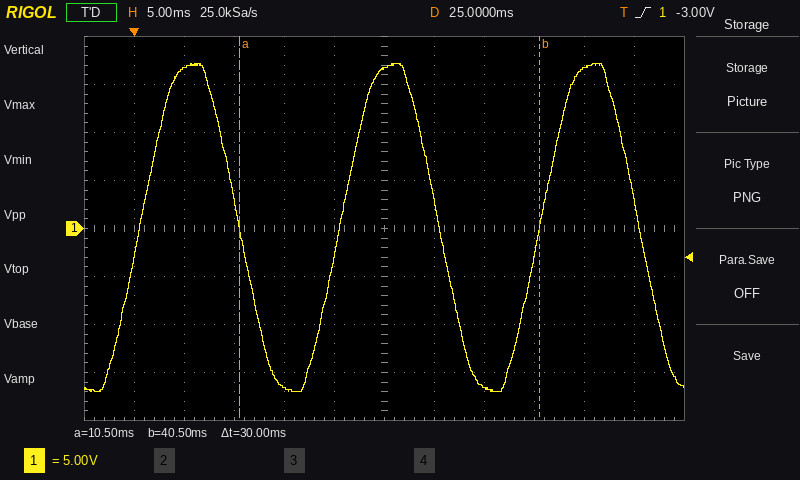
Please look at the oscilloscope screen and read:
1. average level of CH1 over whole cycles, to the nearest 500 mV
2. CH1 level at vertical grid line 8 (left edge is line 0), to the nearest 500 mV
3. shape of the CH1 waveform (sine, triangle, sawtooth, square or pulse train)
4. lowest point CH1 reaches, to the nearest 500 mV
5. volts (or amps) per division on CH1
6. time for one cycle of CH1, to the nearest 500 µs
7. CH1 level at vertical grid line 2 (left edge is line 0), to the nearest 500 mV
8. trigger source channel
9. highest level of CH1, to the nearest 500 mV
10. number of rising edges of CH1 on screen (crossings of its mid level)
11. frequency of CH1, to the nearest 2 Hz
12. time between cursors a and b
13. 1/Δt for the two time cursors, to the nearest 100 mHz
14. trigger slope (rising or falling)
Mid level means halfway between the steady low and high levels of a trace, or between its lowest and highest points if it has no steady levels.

0.0 V
-16.5 V
sine
-17.0 V
5 V
20.0 ms
17.0 V
CH1
17.0 V
3
50 Hz
30 ms
33.3 Hz
rising
